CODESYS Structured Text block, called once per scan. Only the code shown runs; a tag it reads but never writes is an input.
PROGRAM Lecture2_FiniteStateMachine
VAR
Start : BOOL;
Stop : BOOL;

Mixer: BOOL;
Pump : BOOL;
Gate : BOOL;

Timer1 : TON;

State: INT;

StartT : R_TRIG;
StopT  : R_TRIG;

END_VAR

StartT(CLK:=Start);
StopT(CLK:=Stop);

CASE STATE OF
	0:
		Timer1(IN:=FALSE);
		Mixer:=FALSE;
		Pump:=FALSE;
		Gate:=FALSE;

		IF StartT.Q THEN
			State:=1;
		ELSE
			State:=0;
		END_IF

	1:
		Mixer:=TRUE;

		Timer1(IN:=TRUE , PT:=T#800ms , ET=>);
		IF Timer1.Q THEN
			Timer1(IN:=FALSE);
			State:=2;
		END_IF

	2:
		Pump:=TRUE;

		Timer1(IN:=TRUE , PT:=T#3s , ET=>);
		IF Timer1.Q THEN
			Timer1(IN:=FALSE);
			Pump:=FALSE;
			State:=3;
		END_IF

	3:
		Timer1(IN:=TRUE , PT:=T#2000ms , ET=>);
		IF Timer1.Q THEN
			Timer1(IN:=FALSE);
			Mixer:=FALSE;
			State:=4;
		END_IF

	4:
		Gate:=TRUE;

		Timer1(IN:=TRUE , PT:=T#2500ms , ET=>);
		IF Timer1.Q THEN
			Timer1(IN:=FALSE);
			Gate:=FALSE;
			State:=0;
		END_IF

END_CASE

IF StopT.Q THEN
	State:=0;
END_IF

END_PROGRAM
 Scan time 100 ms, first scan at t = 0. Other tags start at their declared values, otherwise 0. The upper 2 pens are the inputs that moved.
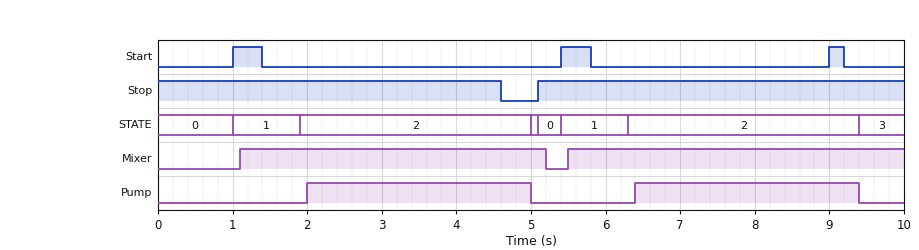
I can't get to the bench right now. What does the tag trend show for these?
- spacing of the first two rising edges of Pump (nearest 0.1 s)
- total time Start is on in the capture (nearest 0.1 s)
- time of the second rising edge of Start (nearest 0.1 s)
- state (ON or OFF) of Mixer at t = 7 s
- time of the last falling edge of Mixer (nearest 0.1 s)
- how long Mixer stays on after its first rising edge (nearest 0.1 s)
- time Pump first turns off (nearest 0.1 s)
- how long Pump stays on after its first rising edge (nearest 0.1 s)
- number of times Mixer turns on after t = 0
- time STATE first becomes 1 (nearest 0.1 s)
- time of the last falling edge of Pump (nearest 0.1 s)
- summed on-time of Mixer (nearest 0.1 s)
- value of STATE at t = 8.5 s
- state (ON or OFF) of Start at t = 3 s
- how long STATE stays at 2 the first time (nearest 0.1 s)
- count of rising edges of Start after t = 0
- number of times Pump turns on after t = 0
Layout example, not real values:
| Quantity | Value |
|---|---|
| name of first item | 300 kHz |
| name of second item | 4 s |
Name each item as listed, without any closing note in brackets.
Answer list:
| Quantity | Value |
|---|---|
| spacing of the first two rising edges of Pump | 4.4 s |
| total time Start is on in the capture | 1.0 s |
| time of the second rising edge of Start | 5.4 s |
| state (ON or OFF) of Mixer at t = 7 s | ON |
| time of the last falling edge of Mixer | 5.2 s |
| how long Mixer stays on after its first rising edge | 4.1 s |
| time Pump first turns off | 5.0 s |
| how long Pump stays on after its first rising edge | 3.0 s |
| number of times Mixer turns on after t = 0 | 2 |
| time STATE first becomes 1 | 1.0 s |
| time of the last falling edge of Pump | 9.4 s |
| summed on-time of Mixer | 8.6 s |
| value of STATE at t = 8.5 s | 2 |
| state (ON or OFF) of Start at t = 3 s | OFF |
| how long STATE stays at 2 the first time | 3.1 s |
| count of rising edges of Start after t = 0 | 3 |
| number of times Pump turns on after t = 0 | 2 |
